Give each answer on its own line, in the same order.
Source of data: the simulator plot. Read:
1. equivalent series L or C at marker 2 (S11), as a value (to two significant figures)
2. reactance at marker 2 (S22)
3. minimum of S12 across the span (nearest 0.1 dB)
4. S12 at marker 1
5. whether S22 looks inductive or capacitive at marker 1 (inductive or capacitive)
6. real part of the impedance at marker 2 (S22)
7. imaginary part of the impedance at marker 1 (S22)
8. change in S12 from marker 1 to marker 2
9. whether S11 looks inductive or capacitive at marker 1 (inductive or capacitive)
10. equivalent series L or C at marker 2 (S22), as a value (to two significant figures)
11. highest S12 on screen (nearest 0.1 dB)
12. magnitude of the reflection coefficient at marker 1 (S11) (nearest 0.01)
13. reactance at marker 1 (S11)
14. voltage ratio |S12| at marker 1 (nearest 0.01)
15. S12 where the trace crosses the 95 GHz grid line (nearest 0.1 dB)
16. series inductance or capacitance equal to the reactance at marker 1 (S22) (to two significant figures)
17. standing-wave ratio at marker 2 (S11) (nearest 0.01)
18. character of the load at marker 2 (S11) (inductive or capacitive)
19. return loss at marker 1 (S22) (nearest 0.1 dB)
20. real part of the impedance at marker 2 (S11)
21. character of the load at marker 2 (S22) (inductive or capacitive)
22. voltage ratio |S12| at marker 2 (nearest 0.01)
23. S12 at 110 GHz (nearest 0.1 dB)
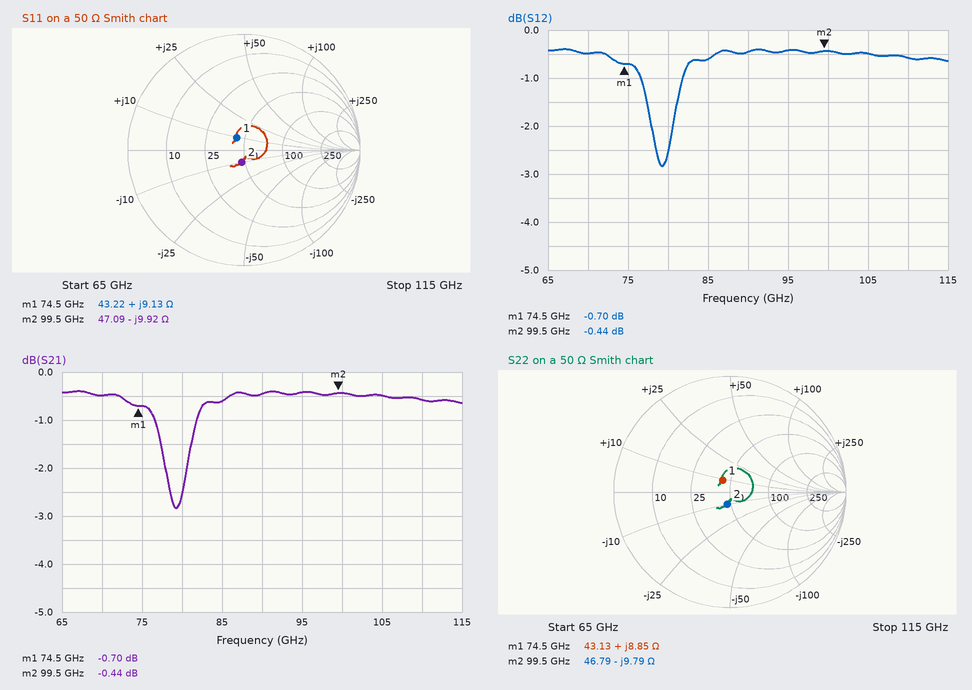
160 fF
-9.79 Ω
-2.8 dB
-0.70 dB
inductive
46.79 Ω
+8.85 Ω
0.26 dB
inductive
160 fF
-0.4 dB
0.12
+9.13 Ω
0.92
-0.4 dB
19 pH
1.24
capacitive
18.4 dB
47.09 Ω
capacitive
0.95
-0.6 dB
